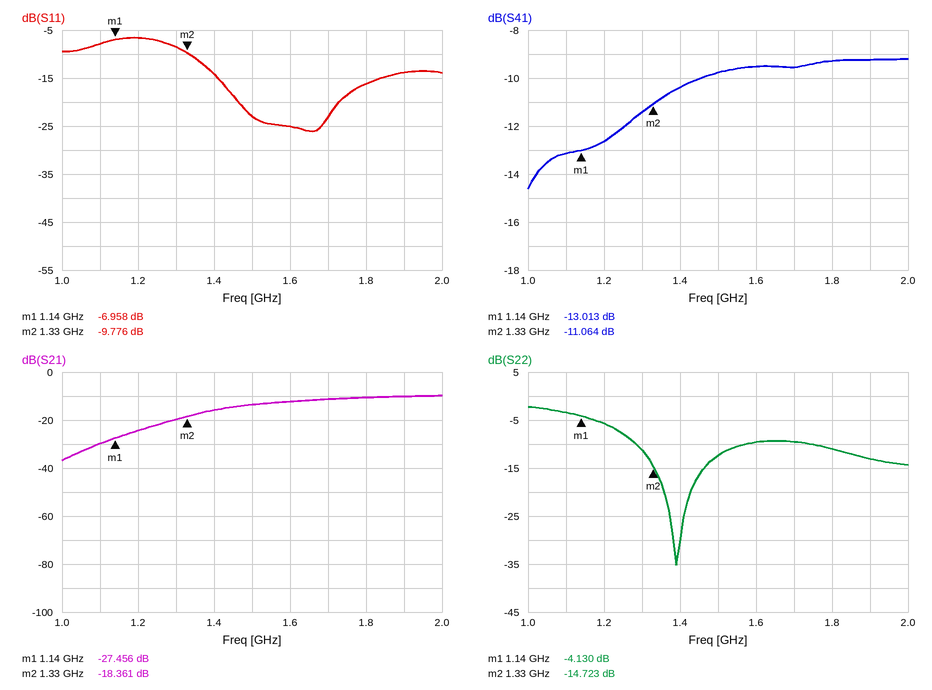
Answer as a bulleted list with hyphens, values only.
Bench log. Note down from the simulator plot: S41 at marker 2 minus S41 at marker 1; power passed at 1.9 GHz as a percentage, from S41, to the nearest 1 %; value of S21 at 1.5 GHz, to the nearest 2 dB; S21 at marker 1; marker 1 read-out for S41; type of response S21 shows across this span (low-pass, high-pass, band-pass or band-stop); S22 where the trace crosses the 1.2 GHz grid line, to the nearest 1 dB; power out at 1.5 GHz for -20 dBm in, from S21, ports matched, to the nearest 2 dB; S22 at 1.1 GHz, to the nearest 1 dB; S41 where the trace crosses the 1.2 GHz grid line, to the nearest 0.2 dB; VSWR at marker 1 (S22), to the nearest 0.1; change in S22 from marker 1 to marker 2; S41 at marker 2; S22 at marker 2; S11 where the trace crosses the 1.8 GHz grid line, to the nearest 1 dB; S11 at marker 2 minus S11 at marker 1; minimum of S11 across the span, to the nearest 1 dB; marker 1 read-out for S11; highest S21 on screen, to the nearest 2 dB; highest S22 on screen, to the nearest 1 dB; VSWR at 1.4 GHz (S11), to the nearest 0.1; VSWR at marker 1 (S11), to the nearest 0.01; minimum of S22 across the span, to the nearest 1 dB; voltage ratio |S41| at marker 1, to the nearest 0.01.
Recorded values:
- 1.949 dB
- 12 %
- -14 dB
- -27.456 dB
- -13.013 dB
- high-pass
- -6 dB
- -34 dBm
- -3 dB
- -12.6 dB
- 4.3
- -10.593 dB
- -11.064 dB
- -14.723 dB
- -16 dB
- -2.818 dB
- -26 dB
- -6.958 dB
- -10 dB
- -2 dB
- 1.5
- 2.63
- -35 dB
- 0.22
